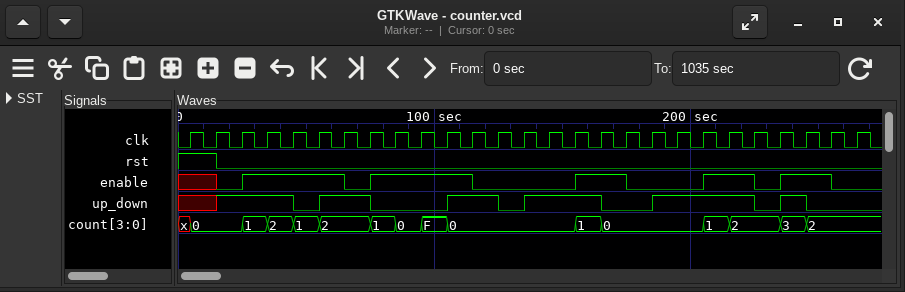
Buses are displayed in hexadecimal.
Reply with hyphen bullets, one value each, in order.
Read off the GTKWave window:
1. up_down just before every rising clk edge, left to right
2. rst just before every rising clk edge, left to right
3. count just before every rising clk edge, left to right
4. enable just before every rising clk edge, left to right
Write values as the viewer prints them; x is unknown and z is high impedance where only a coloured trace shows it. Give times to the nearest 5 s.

- x x 1 1 1 0 1 1 0 0 0 1 1 0 1 1 1 0 0 1 1 1 1 0 1 0 0
- 1 1 0 0 0 0 0 0 0 0 0 0 0 0 0 0 0 0 0 0 0 0 0 0 0 0 0
- x, 0, 0, 1, 2, 1, 2, 2, 1, 0, F, 0, 0, 0, 0, 0, 1, 0, 0, 0, 0, 1, 2, 2, 3, 2, 2
- x x 0 1 1 1 1 0 1 1 1 1 0 0 0 0 1 1 0 0 0 1 1 0 1 1 0
